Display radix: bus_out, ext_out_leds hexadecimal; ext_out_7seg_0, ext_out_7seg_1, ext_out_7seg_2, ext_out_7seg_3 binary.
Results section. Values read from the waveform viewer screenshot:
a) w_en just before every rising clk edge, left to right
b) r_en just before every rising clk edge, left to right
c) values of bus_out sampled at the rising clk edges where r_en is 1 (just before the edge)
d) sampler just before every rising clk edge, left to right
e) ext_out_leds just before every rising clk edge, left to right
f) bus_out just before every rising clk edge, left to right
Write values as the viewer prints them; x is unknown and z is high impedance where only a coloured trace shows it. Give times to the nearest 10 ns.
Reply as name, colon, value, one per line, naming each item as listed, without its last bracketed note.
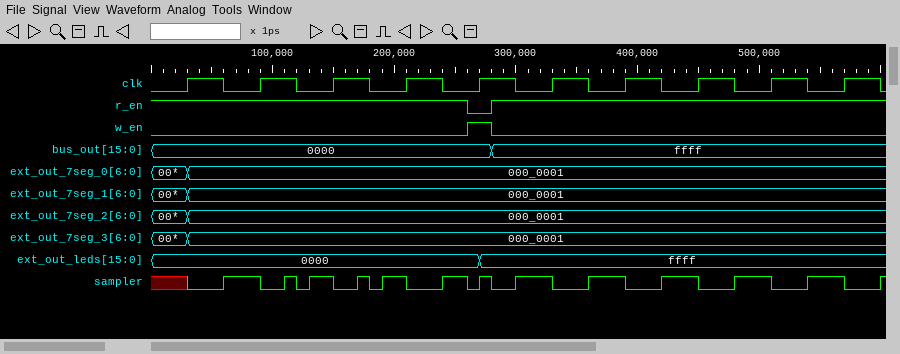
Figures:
w_en just before every rising clk edge, left to right: 0 0 0 0 1 0 0 0 0 0
r_en just before every rising clk edge, left to right: 1 1 1 1 0 1 1 1 1 1
values of bus_out sampled at the rising clk edges where r_en is 1: 0000, 0000, 0000, 0000, ffff, ffff, ffff, ffff, ffff
sampler just before every rising clk edge, left to right: x 1 1 1 0 1 1 1 1 1
ext_out_leds just before every rising clk edge, left to right: 0000, 0000, 0000, 0000, 0000, ffff, ffff, ffff, ffff, ffff
bus_out just before every rising clk edge, left to right: 0000, 0000, 0000, 0000, 0000, ffff, ffff, ffff, ffff, ffff
